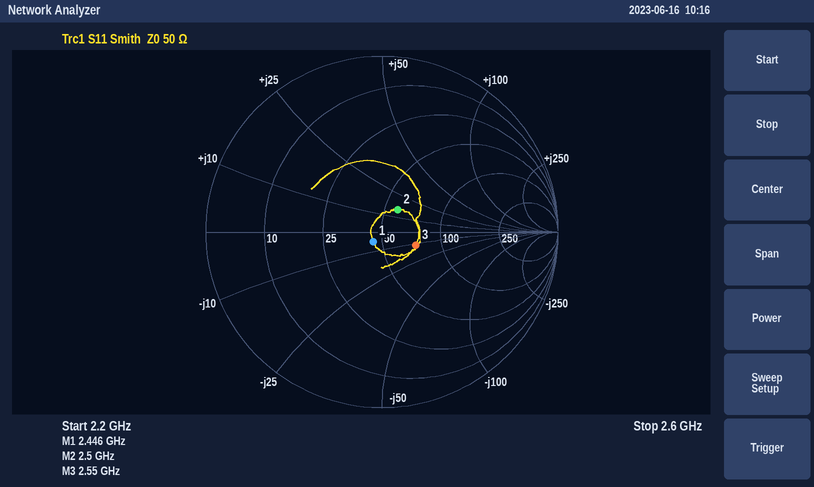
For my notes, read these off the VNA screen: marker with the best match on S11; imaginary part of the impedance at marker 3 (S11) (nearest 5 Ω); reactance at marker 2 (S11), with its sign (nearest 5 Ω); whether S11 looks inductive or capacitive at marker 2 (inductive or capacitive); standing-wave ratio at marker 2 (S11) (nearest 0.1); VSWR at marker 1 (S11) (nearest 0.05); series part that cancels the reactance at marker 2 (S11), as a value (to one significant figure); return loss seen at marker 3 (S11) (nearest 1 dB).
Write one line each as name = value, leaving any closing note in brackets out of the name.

marker with the best match on S11 = marker 1
imaginary part of the impedance at marker 3 (S11) = -10 Ω
reactance at marker 2 (S11), with its sign = +15 Ω
whether S11 looks inductive or capacitive at marker 2 = inductive
standing-wave ratio at marker 2 (S11) = 1.4
VSWR at marker 1 (S11) = 1.15
series part that cancels the reactance at marker 2 (S11), as a value = 4 pF
return loss seen at marker 3 (S11) = 14 dB
